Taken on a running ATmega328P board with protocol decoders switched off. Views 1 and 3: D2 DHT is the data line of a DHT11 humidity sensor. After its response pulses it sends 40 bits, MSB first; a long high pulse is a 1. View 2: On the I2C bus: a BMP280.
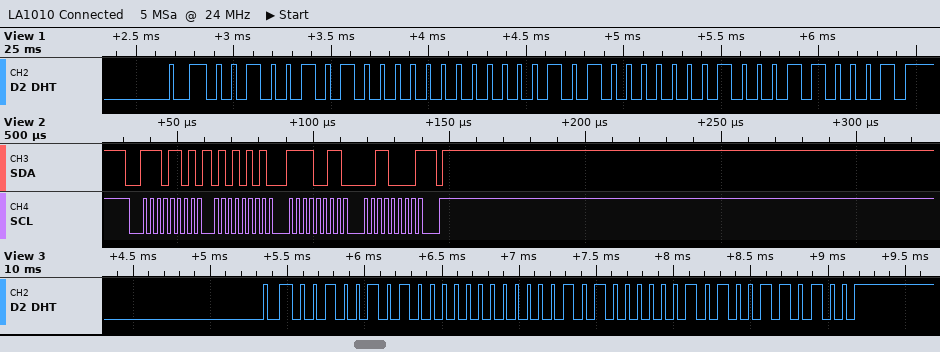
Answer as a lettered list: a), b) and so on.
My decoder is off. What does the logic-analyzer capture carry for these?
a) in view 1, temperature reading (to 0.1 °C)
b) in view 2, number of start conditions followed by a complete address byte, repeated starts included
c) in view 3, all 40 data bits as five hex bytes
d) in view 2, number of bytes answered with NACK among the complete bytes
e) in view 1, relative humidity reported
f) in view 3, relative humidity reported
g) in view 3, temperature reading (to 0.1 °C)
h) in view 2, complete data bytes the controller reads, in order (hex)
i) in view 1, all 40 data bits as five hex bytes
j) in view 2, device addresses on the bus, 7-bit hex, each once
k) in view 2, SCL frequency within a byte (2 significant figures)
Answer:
a) 10.2 °C
b) 1
c) 25 00 0A 05 34
d) 1
e) 37 %
f) 37 %
g) 10.5 °C
h) 55 F3 30
i) 25 00 0A 02 31
j) 0x76
k) 400 kHz
